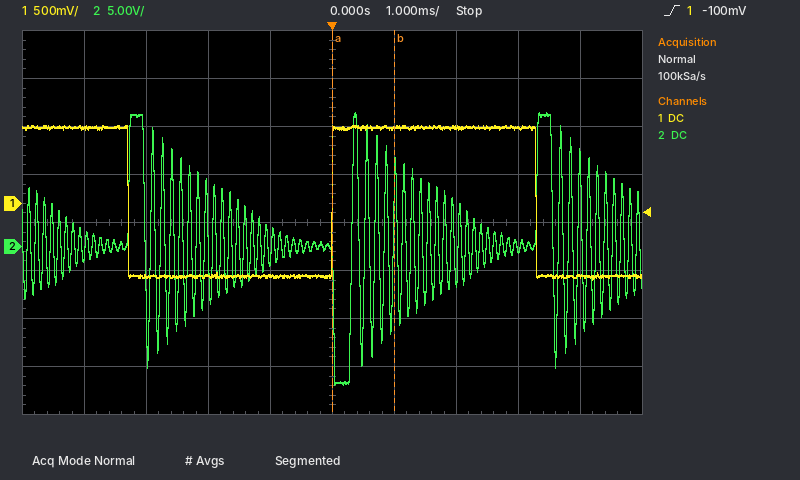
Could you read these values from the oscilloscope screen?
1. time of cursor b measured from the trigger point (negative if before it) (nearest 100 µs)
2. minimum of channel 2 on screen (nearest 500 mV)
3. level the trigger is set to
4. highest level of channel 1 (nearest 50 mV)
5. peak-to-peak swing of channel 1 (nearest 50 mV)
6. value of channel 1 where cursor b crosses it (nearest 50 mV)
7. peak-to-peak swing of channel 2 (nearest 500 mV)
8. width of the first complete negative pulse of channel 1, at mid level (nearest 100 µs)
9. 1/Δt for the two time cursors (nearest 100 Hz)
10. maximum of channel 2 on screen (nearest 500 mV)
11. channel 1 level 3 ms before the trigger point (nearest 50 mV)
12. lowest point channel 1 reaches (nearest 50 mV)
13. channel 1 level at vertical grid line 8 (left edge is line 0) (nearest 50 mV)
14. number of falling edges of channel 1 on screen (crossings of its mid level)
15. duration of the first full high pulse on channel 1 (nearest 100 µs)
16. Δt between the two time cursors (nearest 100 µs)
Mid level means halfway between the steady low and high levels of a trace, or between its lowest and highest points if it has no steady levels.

+1.0 ms
-14.5 V
-100 mV
800 mV
1.60 V
800 mV
28.5 V
3.3 ms
1.0 kHz
14.0 V
-750 mV
-800 mV
800 mV
2
3.3 ms
1.0 ms
